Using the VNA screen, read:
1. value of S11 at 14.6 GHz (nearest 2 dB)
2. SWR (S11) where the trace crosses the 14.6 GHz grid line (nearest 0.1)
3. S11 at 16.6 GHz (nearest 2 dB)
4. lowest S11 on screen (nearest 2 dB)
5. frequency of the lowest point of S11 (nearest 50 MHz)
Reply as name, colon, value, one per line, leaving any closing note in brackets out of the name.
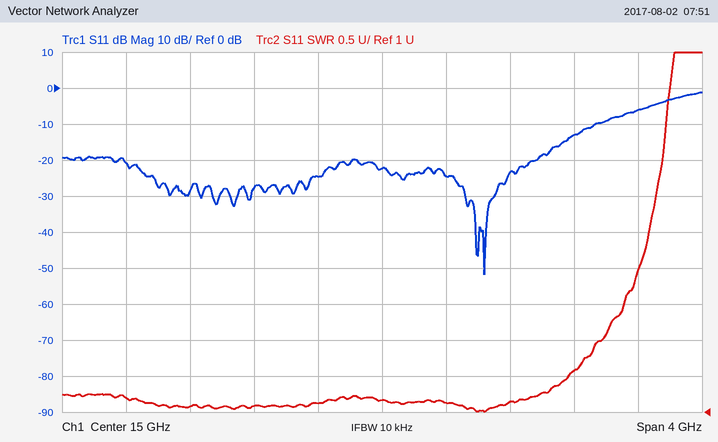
value of S11 at 14.6 GHz: -24 dB
SWR (S11) where the trace crosses the 14.6 GHz grid line: 1.1
S11 at 16.6 GHz: -6 dB
lowest S11 on screen: -52 dB
frequency of the lowest point of S11: 15.65 GHz
